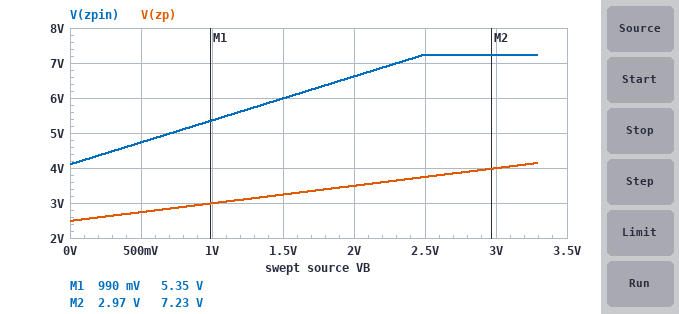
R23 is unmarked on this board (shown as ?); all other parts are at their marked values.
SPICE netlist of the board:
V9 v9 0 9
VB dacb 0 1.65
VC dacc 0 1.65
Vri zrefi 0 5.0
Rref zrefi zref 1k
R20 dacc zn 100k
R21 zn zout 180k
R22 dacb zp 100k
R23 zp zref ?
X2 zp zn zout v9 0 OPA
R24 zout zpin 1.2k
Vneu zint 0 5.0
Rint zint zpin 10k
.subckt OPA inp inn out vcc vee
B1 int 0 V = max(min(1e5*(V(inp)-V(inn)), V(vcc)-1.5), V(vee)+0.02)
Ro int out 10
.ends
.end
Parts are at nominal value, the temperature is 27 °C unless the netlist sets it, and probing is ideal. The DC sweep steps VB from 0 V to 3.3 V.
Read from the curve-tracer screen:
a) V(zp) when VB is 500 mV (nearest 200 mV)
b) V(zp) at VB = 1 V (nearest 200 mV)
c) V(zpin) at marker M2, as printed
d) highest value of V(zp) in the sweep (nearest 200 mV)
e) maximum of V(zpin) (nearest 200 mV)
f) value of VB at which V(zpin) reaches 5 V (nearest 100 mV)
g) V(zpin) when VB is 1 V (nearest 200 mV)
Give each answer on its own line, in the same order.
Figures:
2.8 V
3.0 V
7.23 V
4.2 V
7.2 V
700 mV
5.4 V
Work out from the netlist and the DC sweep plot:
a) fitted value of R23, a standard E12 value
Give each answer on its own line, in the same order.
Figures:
100 kΩ
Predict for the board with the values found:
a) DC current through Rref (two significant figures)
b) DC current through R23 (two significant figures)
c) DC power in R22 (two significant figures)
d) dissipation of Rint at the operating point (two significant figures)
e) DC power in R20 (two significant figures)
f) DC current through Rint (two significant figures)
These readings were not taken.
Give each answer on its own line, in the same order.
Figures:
17 µA
17 µA
28 µW
140 µW
28 µW
120 µA
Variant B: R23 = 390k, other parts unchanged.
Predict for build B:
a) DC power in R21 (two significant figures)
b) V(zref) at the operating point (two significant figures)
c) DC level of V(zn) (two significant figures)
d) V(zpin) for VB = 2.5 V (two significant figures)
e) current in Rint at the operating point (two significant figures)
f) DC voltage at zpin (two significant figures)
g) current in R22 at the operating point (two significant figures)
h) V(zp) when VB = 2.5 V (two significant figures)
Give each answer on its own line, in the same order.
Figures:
8.4 µW
5.0 V
2.3 V
5.4 V
130 µA
3.7 V
6.8 µA
3.0 V
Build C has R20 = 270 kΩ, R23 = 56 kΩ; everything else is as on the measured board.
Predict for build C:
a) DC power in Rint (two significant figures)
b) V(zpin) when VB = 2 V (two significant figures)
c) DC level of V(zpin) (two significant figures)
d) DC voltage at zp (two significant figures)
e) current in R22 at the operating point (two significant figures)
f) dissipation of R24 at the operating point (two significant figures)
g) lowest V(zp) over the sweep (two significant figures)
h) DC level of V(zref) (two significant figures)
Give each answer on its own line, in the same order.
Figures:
3.4 µW
5.4 V
5.2 V
3.8 V
21 µA
410 nW
3.2 V
5.0 V
